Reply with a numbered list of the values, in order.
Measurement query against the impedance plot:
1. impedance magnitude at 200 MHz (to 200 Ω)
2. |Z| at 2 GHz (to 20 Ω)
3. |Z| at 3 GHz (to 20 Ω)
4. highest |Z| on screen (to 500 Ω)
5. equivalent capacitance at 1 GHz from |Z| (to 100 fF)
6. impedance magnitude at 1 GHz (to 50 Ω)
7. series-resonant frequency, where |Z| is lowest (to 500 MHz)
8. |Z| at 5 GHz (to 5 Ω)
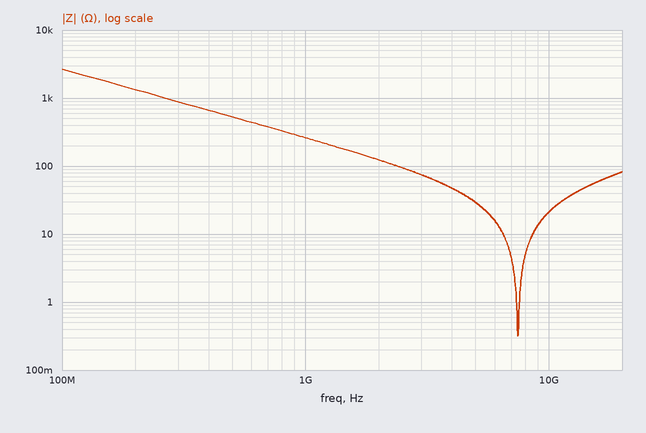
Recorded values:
1. 1.4 kΩ
2. 120 Ω
3. 80 Ω
4. 2.5 kΩ
5. 600 fF
6. 250 Ω
7. 7.5 GHz
8. 30 Ω
